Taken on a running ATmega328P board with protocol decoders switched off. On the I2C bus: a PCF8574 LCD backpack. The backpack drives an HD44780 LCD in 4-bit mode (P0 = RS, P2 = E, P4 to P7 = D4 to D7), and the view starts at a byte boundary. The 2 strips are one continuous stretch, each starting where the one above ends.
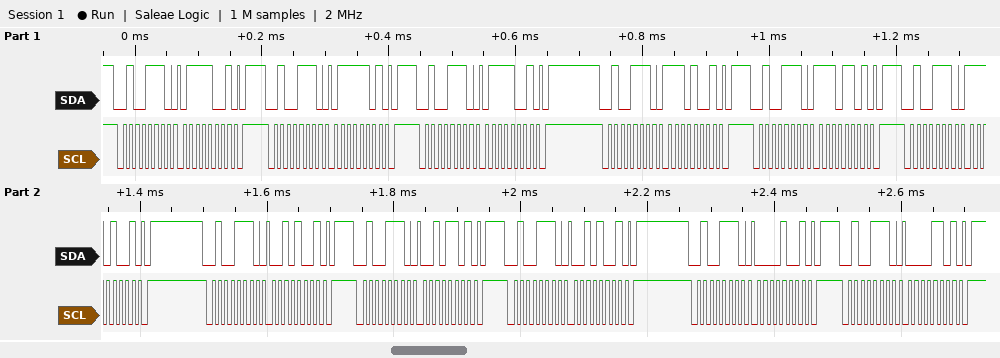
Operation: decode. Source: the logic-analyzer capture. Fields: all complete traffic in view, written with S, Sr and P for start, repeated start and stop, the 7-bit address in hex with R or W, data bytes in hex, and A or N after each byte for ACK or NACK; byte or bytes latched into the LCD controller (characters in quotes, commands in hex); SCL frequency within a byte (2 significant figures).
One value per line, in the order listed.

S 27W A 79 A P S 27W A 7D A P S 27W A 79 A P S 27W A E9 A P S 27W A ED A P S 27W A E9 A P S 27W A 29 A P S 27W A 2D A P S 27W A 29 A P S 27W A 09 A P S 27W A 0D A P
data 0x7E
100 kHz
